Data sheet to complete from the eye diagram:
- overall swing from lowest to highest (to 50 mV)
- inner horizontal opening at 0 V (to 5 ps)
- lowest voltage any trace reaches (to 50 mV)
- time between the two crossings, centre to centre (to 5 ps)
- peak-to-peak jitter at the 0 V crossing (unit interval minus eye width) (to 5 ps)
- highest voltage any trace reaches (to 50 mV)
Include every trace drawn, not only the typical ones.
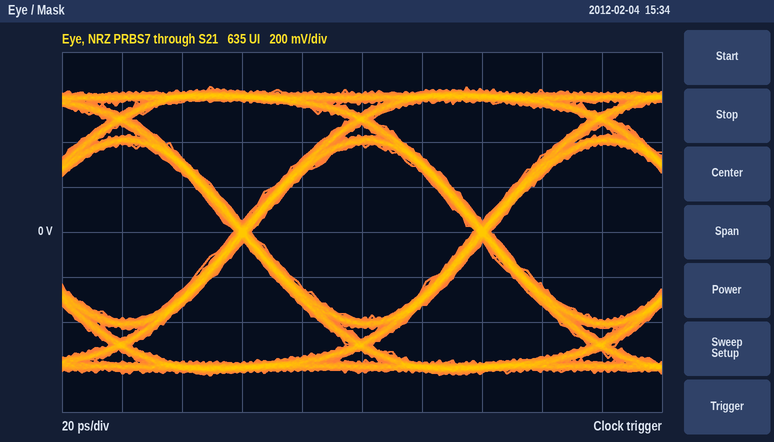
1.30 V
75 ps
-650 mV
80 ps
5 ps
650 mV
